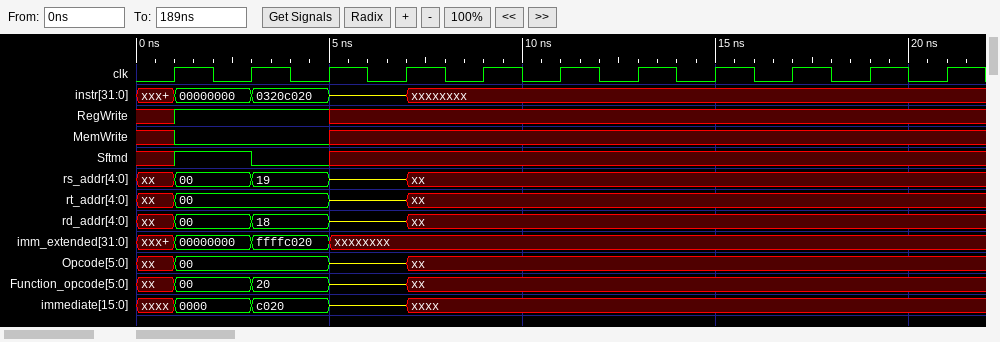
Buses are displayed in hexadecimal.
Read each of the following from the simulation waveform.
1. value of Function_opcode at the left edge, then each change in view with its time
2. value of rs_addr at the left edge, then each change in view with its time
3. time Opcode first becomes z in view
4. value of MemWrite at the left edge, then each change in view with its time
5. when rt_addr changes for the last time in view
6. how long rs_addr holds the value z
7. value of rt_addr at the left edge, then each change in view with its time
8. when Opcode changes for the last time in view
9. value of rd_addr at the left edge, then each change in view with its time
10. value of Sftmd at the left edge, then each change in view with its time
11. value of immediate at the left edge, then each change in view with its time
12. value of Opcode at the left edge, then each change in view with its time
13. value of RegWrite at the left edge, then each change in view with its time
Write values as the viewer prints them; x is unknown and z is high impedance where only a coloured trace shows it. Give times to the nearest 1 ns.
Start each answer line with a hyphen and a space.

- xx, 00 at 1 ns, 20 at 3 ns, z at 5 ns, xx at 7 ns
- xx, 00 at 1 ns, 19 at 3 ns, z at 5 ns, xx at 7 ns
- 5 ns
- x, 0 at 1 ns, x at 5 ns
- 7 ns
- 2 ns
- xx, 00 at 1 ns, z at 5 ns, xx at 7 ns
- 7 ns
- xx, 00 at 1 ns, 18 at 3 ns, z at 5 ns, xx at 7 ns
- x, 1 at 1 ns, 0 at 3 ns, x at 5 ns
- xxxx, 0000 at 1 ns, c020 at 3 ns, z at 5 ns, xxxx at 7 ns
- xx, 00 at 1 ns, z at 5 ns, xx at 7 ns
- x, 1 at 1 ns, x at 5 ns
